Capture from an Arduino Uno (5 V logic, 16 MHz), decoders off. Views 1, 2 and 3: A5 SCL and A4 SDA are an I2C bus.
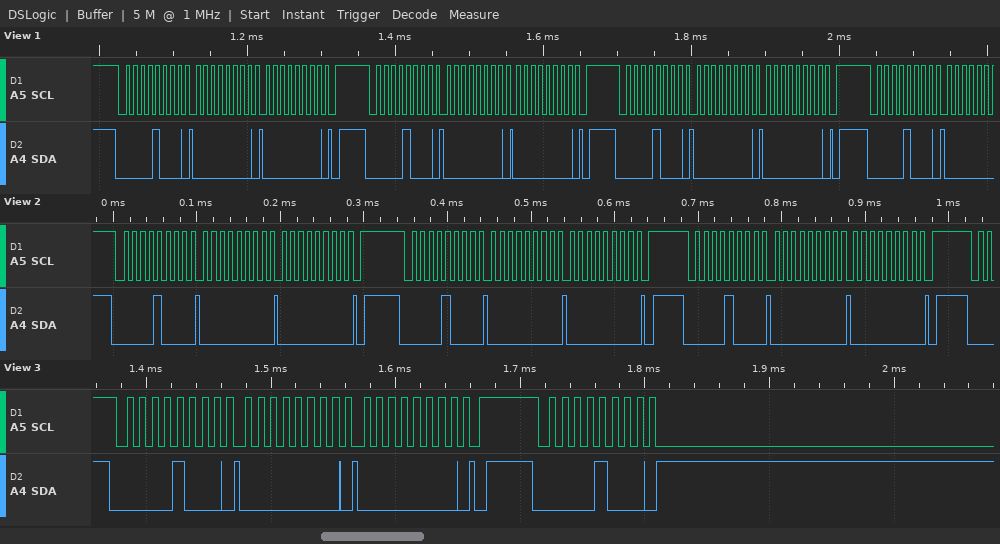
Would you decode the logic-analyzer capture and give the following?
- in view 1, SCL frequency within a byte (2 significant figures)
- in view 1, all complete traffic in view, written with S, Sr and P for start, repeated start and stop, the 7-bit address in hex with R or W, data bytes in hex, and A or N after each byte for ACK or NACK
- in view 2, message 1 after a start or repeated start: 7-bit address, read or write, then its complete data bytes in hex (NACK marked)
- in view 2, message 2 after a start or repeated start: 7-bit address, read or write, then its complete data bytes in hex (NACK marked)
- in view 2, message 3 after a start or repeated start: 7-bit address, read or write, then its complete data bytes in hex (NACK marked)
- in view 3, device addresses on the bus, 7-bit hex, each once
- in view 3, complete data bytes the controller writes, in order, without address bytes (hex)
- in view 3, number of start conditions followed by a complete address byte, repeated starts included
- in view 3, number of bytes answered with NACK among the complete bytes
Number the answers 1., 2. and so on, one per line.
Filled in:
1. 100 kHz
2. S 04W A 00 A 00 A P S 04W A 00 A 00 A P S 04W A 00 A 00 A P S 04W A
3. 0x04 write: 00 00
4. 0x04 write: 00 00
5. 0x04 write: 00 00
6. 0x04
7. 00 00
8. 2
9. 0
